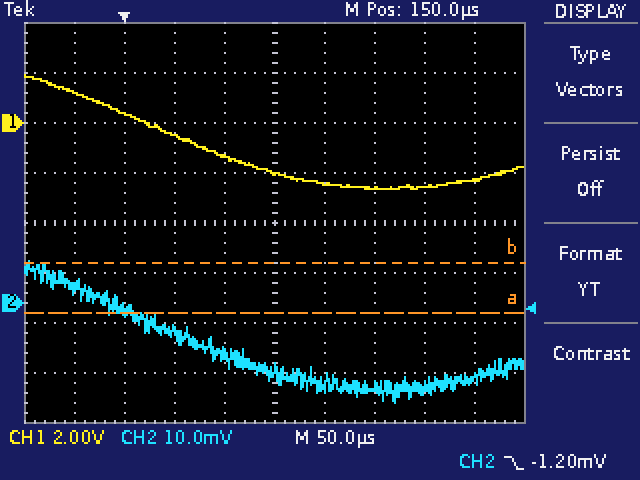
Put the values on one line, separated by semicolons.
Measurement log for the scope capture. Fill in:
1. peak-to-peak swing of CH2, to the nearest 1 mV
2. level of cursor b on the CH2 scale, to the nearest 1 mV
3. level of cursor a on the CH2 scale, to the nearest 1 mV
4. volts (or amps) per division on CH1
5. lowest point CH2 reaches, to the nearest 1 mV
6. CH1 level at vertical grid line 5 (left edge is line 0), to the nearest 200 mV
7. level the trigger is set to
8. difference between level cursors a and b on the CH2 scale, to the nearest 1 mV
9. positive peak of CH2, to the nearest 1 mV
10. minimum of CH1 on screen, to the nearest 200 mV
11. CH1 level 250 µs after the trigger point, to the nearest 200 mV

28 mV; 8 mV; -2 mV; 2 V; -20 mV; -2.0 V; -1.20 mV; 10 mV; 8 mV; -2.6 V; -2.6 V
